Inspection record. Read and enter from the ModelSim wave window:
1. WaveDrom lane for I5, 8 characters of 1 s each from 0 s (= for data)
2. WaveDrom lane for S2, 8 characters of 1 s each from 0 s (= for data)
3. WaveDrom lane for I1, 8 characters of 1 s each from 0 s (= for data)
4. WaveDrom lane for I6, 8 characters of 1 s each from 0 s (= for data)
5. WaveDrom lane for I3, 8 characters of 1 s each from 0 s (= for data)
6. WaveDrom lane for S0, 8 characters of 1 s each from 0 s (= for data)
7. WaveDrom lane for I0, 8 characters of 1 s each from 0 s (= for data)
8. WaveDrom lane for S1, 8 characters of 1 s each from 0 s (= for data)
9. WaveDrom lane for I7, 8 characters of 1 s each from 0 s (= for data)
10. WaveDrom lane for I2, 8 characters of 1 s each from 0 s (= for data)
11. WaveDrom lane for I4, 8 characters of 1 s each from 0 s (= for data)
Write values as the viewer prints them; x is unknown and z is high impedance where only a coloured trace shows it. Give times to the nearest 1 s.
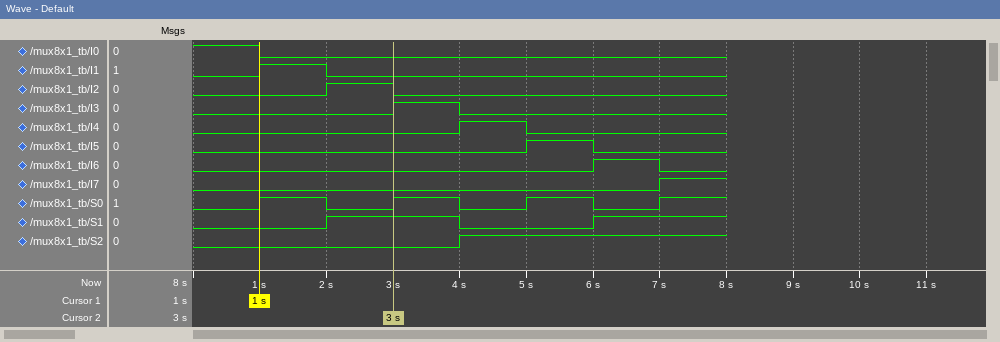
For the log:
{name: 'I5', wave: '0....10.'}
{name: 'S2', wave: '0...1...'}
{name: 'I1', wave: '010.....'}
{name: 'I6', wave: '0.....10'}
{name: 'I3', wave: '0..10...'}
{name: 'S0', wave: '01010101'}
{name: 'I0', wave: '10......'}
{name: 'S1', wave: '0.1.0.1.'}
{name: 'I7', wave: '0......1'}
{name: 'I2', wave: '0.10....'}
{name: 'I4', wave: '0...10..'}
